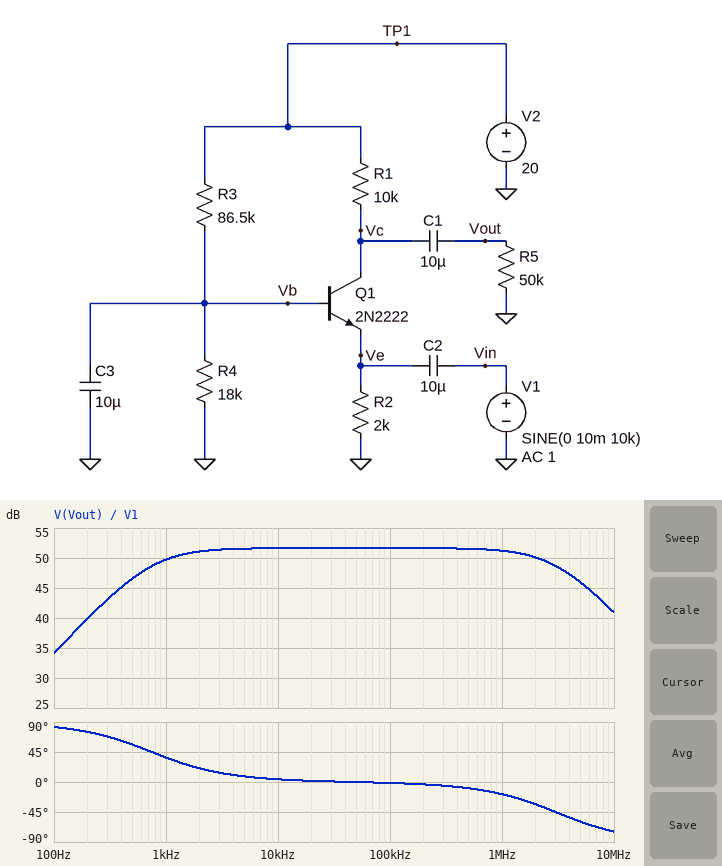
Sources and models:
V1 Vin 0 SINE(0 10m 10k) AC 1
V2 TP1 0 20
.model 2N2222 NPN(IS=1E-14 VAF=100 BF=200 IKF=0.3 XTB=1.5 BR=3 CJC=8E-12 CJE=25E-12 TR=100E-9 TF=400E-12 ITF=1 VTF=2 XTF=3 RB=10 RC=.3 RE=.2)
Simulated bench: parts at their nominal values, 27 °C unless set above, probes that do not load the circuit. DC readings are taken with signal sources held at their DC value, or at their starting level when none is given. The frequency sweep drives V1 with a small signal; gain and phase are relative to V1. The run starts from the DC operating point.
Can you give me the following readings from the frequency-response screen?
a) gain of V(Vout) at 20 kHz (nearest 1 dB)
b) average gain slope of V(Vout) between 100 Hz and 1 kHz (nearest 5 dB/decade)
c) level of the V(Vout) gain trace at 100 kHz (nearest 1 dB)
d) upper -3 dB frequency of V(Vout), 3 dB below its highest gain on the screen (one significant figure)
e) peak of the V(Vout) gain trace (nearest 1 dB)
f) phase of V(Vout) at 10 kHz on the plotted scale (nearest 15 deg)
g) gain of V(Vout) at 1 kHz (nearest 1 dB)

52 dB
15 dB/decade
52 dB
3 MHz
52 dB
0 deg
50 dB
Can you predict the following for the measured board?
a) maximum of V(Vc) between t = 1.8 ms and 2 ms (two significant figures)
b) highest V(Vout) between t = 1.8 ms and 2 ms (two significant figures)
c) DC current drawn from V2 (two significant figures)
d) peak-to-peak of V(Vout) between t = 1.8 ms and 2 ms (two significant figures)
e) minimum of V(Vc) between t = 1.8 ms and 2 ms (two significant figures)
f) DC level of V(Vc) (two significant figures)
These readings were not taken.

10 V
3.5 V
1.5 mA
7.3 V
2.8 V
6.6 V
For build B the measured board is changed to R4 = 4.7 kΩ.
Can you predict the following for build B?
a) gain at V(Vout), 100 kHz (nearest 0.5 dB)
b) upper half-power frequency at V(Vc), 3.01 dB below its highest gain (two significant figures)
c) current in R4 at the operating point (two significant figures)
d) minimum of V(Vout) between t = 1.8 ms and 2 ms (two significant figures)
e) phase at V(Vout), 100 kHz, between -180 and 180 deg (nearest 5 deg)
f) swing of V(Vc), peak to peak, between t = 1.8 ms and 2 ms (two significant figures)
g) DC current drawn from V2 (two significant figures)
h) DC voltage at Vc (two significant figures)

36.5 dB
6.3 MHz
220 µA
-730 mV
0 deg
1.3 V
430 µA
18 V
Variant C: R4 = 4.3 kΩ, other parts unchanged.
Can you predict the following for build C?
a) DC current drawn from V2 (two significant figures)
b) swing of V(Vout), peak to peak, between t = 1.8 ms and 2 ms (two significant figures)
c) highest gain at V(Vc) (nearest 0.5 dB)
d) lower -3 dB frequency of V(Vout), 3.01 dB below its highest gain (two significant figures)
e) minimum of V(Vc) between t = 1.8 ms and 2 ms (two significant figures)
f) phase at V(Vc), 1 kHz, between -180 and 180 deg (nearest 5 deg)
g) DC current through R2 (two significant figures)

390 µA
1.1 V
34.5 dB
110 Hz
18 V
5 deg
170 µA
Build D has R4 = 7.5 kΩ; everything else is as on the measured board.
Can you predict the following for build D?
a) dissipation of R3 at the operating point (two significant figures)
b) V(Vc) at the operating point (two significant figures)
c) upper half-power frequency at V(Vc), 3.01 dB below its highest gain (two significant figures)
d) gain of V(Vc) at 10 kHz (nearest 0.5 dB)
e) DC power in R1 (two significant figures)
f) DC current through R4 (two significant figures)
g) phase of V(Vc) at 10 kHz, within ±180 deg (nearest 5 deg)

3.9 mW
15 V
5.5 MHz
43.5 dB
2.2 mW
210 µA
0 deg
